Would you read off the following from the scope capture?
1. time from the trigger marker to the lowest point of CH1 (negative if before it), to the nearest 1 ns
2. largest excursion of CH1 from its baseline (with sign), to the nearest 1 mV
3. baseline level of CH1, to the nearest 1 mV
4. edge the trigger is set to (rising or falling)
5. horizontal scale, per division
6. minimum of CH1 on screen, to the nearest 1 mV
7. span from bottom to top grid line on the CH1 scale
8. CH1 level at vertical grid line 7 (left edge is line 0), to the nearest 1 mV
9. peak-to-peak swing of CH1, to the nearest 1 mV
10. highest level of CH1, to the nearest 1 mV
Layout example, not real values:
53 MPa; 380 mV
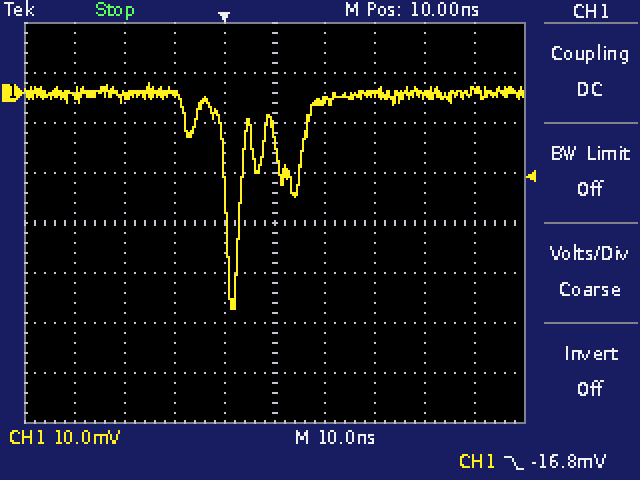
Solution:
+2 ns; -43 mV; 0 mV; falling; 10 ns; -43 mV; 80 mV; 0 mV; 45 mV; 2 mV
